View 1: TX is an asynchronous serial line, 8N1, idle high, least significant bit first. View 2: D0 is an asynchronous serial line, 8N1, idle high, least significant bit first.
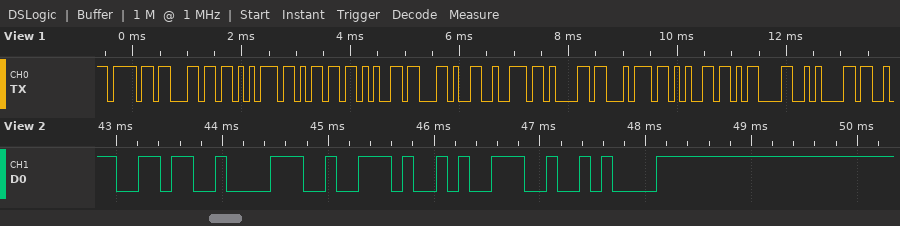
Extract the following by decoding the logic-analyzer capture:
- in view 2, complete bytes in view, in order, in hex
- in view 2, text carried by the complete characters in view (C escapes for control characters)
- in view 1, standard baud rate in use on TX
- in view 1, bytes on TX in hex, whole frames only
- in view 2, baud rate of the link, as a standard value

36 38 2E 39 0A
"68.9\n"
9600 baud
6F 6C 75 6D 65 2C 72 61 74 65 0D 0A
9600 baud
